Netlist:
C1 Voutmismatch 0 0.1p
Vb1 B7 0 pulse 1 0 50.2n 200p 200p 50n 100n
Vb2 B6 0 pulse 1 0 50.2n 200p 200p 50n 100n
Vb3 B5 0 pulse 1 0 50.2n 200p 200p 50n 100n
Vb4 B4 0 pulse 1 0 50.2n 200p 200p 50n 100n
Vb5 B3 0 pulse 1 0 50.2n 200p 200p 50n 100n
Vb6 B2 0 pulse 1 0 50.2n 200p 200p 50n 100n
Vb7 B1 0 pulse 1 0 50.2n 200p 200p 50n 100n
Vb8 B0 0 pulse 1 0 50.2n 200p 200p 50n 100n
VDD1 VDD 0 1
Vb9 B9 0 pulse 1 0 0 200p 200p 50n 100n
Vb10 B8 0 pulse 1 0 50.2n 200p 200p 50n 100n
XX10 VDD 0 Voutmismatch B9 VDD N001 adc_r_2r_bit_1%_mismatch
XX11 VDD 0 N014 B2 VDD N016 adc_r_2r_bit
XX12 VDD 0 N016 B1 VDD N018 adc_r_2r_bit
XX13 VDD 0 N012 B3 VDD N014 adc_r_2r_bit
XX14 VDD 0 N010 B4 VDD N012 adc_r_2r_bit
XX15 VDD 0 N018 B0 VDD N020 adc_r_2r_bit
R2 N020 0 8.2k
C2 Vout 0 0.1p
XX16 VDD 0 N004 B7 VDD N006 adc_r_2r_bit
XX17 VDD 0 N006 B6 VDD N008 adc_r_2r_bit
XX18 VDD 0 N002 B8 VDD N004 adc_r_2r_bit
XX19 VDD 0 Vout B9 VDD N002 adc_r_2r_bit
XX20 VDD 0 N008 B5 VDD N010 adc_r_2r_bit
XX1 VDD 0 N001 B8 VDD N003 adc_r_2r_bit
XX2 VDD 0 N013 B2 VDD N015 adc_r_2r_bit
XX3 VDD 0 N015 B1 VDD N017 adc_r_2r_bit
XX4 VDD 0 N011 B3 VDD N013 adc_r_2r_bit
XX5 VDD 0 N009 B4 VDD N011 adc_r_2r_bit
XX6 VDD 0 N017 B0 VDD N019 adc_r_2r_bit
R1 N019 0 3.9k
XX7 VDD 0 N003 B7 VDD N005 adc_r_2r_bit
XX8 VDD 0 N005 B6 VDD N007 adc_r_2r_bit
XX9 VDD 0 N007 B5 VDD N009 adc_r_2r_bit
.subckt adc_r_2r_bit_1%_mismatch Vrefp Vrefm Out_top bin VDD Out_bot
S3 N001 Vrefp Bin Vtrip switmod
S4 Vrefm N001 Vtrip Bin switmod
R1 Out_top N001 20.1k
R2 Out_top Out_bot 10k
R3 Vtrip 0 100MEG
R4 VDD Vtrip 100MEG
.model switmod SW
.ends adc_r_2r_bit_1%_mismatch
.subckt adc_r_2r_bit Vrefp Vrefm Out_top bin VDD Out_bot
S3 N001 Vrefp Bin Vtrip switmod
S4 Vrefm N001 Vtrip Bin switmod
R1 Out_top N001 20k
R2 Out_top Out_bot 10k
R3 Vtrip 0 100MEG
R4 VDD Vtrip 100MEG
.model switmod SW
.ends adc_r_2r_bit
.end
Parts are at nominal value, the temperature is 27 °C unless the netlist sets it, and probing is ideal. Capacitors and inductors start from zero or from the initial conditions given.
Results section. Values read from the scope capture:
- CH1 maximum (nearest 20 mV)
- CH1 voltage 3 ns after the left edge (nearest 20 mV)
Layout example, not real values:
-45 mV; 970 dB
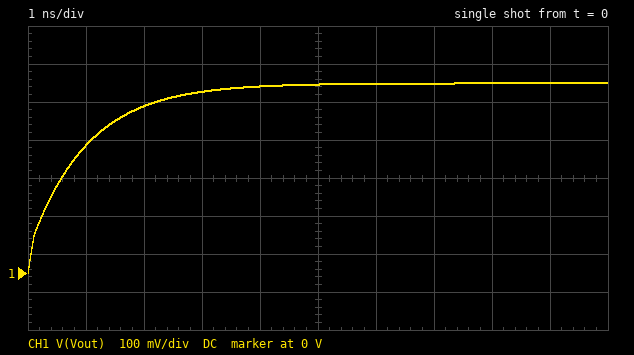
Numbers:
500 mV; 480 mV
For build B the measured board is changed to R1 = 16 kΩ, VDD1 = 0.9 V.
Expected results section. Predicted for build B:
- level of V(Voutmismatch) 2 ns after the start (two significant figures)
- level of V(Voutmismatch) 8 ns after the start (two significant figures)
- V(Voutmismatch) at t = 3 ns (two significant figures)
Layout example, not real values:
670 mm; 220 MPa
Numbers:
400 mV; 450 mV; 430 mV
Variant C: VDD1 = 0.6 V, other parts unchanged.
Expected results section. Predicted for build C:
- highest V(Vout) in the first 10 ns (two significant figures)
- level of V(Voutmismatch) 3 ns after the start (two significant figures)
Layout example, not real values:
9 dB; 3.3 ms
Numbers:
300 mV; 290 mV
